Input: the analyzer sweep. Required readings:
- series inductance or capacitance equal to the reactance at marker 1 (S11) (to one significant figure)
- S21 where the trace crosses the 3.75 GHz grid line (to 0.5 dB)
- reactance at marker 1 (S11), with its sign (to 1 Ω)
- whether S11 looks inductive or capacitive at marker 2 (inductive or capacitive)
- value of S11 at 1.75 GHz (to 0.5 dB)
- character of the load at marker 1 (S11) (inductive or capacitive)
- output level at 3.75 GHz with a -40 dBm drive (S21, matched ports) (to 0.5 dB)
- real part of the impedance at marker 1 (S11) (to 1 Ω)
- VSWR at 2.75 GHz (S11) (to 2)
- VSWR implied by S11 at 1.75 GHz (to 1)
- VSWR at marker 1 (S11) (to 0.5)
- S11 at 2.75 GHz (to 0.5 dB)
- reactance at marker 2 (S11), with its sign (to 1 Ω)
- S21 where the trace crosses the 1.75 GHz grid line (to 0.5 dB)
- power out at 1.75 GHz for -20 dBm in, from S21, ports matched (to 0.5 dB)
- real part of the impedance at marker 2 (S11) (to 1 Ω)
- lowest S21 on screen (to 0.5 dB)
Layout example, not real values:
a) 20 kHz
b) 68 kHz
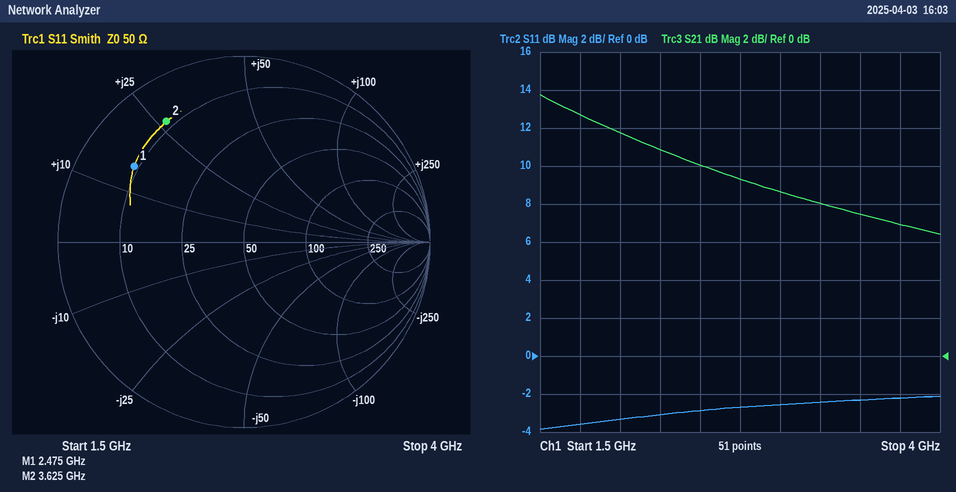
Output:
a) 1.0 nH
b) 7.0 dB
c) +15 Ω
d) inductive
e) -3.5 dB
f) inductive
g) -33.0 dBm
h) 9 Ω
i) 6
j) 5
k) 6.0
l) -2.5 dB
m) +27 Ω
n) 12.5 dB
o) -7.5 dBm
p) 8 Ω
q) 6.5 dB
